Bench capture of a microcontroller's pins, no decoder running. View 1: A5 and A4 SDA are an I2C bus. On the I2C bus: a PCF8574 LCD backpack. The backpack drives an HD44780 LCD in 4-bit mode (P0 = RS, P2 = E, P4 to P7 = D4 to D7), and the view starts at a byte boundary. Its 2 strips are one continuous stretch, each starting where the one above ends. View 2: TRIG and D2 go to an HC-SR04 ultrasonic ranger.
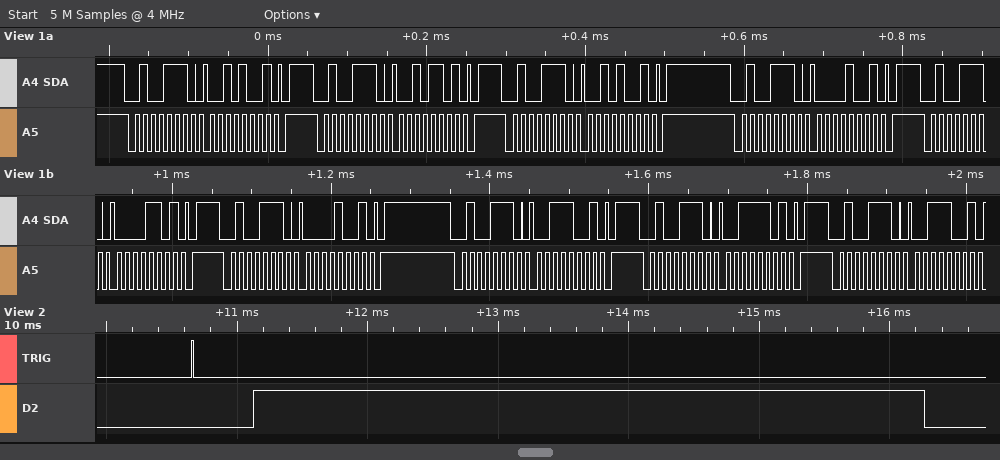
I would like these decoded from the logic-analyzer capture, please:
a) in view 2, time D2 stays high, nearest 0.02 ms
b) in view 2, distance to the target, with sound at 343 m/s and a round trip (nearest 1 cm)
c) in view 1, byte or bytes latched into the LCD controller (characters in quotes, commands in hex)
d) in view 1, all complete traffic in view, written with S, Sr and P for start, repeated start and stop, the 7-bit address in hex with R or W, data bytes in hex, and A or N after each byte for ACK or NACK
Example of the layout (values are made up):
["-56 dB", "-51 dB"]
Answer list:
["5.14 ms", "88 cm", "' '", "S 27W A 29 A P S 27W A 2D A P S 27W A 29 A P S 27W A 09 A P S 27W A 0D A P S 27W A 09 A P S 27W A 39 A P S 27W A 3D A P S 27W A 39 A"]
